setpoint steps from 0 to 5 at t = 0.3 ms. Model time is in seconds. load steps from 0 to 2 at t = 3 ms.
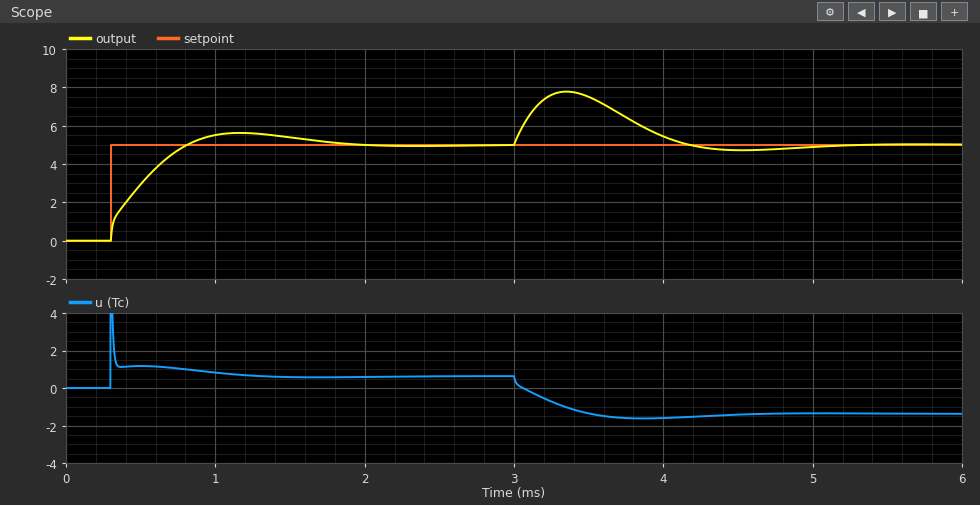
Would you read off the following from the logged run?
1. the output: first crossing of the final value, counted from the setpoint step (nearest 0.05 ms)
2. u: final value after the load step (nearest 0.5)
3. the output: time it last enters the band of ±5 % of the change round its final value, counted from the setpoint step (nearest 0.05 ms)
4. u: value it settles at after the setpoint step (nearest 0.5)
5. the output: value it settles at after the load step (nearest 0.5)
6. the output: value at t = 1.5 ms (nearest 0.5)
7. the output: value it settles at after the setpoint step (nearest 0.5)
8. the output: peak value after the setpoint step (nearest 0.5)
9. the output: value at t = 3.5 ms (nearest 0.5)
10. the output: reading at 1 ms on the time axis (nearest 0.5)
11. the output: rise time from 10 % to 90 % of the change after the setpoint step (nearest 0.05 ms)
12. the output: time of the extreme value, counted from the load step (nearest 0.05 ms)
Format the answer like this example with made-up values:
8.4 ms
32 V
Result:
0.50 ms
-1.5
1.35 ms
0.5
5.0
5.5
5.0
5.5
7.5
5.5
0.40 ms
0.35 ms
